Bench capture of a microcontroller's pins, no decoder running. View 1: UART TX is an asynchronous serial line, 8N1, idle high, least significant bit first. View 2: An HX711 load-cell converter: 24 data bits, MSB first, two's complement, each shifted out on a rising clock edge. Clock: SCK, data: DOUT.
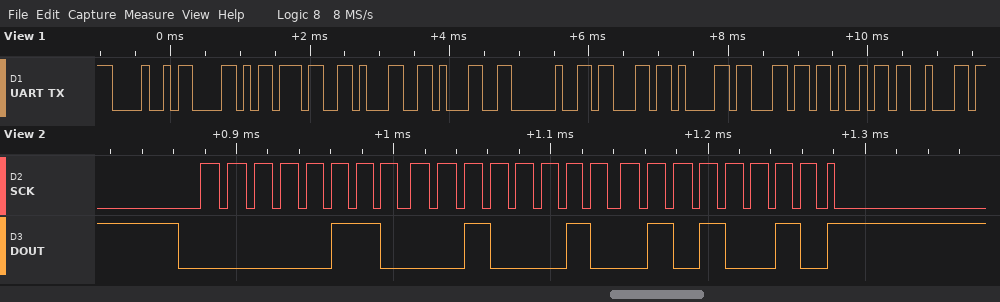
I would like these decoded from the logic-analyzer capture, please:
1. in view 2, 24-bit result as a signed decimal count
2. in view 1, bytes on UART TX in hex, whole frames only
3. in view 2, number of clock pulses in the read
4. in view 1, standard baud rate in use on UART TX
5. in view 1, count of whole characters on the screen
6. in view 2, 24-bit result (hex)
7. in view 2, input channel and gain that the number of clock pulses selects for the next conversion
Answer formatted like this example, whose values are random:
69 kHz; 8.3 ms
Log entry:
402002; 0x48 0x58 0x37 0x31 0x31 0x20 0x63 0x61 0x6C 0x69 0x62; 25; 9600 baud; 11; 0x062252; channel A, gain 128
